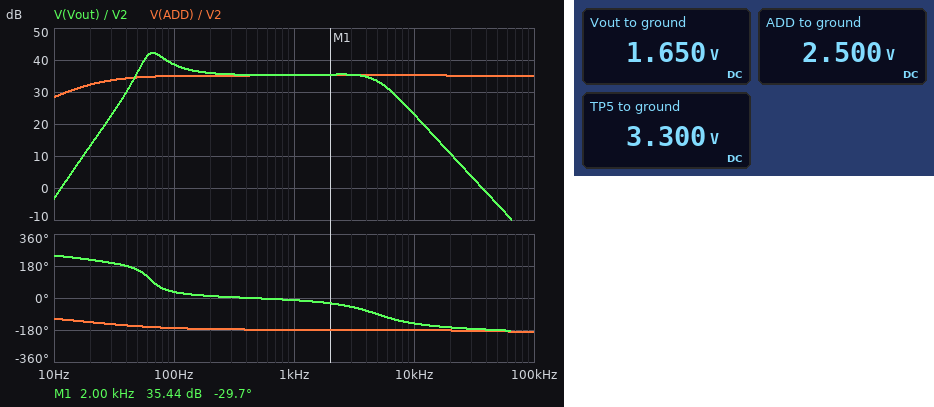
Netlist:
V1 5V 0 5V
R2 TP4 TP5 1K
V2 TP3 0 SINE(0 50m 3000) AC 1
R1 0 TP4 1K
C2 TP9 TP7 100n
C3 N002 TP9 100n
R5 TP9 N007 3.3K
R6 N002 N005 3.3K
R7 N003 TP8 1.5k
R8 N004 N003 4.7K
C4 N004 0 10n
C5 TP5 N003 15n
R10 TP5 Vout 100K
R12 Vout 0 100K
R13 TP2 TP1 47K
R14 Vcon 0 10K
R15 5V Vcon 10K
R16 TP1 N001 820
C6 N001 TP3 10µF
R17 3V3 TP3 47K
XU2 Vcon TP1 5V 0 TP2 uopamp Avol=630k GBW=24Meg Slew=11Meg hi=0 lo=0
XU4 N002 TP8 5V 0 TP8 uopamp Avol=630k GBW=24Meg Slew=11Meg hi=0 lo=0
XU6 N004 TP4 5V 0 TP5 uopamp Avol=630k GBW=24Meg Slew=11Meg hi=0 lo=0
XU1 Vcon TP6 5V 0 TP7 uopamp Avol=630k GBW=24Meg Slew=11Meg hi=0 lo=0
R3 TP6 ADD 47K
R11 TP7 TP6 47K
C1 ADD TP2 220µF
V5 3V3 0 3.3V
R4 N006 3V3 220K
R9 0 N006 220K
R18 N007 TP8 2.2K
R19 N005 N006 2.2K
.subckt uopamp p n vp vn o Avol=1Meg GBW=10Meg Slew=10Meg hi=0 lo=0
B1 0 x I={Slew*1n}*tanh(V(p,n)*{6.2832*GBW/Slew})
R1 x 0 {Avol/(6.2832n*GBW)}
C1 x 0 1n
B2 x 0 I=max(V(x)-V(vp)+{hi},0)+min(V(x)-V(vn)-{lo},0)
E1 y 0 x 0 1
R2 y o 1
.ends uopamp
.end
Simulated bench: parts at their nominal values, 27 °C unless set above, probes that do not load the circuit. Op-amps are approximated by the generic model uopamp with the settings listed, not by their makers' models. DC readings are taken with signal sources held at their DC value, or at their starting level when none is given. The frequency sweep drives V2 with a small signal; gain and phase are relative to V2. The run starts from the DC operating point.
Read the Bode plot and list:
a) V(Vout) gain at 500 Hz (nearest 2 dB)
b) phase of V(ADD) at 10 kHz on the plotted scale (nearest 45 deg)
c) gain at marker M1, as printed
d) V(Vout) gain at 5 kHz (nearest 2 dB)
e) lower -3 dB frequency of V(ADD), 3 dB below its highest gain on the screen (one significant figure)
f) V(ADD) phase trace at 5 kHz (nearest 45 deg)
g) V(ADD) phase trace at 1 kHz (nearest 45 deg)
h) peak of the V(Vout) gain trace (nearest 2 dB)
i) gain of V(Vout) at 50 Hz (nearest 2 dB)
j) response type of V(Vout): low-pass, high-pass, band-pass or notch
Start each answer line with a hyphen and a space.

- 36 dB
- -180 deg
- 35.44 dB
- 34 dB
- 20 Hz
- -180 deg
- -180 deg
- 42 dB
- 36 dB
- band-pass
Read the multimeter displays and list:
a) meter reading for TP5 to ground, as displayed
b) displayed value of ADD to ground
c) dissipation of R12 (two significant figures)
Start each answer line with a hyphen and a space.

- 3.300 V
- 2.500 V
- 27 µW
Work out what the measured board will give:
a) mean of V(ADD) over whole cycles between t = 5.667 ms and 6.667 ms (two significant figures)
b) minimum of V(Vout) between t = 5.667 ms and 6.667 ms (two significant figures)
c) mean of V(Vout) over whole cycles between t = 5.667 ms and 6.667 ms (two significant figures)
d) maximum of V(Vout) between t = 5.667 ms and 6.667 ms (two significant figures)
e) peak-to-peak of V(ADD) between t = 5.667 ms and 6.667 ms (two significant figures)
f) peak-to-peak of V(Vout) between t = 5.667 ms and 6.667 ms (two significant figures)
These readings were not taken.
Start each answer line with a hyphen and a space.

- 2.5 V
- -5.1 mV
- 1.6 V
- 2.5 V
- 5.0 V
- 2.5 V
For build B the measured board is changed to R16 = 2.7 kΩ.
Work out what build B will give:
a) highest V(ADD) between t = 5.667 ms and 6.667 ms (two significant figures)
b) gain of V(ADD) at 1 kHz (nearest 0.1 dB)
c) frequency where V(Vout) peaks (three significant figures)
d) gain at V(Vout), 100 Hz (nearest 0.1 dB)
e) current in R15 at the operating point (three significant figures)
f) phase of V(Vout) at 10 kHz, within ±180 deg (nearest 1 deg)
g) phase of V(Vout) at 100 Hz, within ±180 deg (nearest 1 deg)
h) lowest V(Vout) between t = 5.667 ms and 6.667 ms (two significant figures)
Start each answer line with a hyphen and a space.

- 3.4 V
- 24.8 dB
- 66.4 Hz
- 28.4 dB
- 250 µA
- -142 deg
- 27 deg
- 750 mV
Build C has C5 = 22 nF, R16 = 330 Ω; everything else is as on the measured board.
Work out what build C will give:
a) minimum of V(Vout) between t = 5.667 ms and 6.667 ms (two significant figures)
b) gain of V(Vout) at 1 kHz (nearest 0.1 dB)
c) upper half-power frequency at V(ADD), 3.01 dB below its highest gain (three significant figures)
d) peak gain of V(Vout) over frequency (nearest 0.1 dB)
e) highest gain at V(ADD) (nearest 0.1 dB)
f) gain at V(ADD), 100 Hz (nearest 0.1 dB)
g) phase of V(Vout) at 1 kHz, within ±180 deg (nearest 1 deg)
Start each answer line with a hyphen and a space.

- -5.3 mV
- 43.5 dB
- 167 kHz
- 48.7 dB
- 43.1 dB
- 42.2 dB
- -7 deg
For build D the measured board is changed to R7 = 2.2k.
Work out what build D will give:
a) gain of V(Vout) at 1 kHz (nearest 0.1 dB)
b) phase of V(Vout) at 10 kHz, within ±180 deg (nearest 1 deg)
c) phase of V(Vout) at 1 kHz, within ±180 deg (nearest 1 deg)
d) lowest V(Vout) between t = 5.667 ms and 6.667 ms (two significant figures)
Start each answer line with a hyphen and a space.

- 35.5 dB
- -157 deg
- -11 deg
- -5.2 mV
